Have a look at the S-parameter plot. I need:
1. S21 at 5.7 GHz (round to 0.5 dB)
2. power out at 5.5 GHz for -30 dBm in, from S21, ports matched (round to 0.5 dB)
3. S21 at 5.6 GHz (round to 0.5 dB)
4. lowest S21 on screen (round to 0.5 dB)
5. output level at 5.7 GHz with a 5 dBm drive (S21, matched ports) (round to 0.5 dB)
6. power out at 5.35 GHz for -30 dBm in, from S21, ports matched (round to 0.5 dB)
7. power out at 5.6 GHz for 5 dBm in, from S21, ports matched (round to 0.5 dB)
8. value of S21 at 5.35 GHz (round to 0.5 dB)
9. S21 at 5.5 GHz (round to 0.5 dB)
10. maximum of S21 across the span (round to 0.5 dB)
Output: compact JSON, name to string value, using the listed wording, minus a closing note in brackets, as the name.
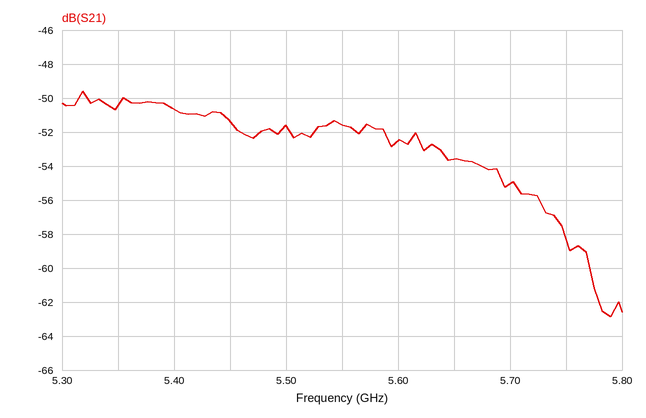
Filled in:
{"S21 at 5.7 GHz": "-55.0 dB", "power out at 5.5 GHz for -30 dBm in, from S21, ports matched": "-81.5 dBm", "S21 at 5.6 GHz": "-52.5 dB", "lowest S21 on screen": "-63.0 dB", "output level at 5.7 GHz with a 5 dBm drive (S21, matched ports)": "-50.0 dBm", "power out at 5.35 GHz for -30 dBm in, from S21, ports matched": "-80.5 dBm", "power out at 5.6 GHz for 5 dBm in, from S21, ports matched": "-47.5 dBm", "value of S21 at 5.35 GHz": "-50.5 dB", "S21 at 5.5 GHz": "-51.5 dB", "maximum of S21 across the span": "-49.5 dB"}
